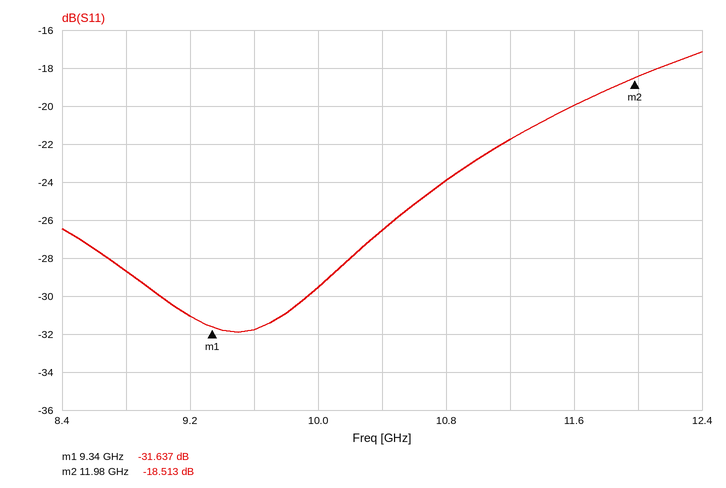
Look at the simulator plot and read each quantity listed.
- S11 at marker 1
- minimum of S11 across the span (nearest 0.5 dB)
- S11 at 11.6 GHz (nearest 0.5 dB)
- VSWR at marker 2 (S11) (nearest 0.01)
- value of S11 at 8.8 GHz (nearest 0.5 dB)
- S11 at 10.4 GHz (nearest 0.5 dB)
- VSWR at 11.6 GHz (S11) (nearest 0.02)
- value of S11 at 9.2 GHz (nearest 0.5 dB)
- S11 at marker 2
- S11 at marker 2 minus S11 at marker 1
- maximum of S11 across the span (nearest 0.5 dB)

-31.637 dB
-32.0 dB
-20.0 dB
1.27
-28.5 dB
-26.5 dB
1.22
-31.0 dB
-18.513 dB
13.124 dB
-17.0 dB
